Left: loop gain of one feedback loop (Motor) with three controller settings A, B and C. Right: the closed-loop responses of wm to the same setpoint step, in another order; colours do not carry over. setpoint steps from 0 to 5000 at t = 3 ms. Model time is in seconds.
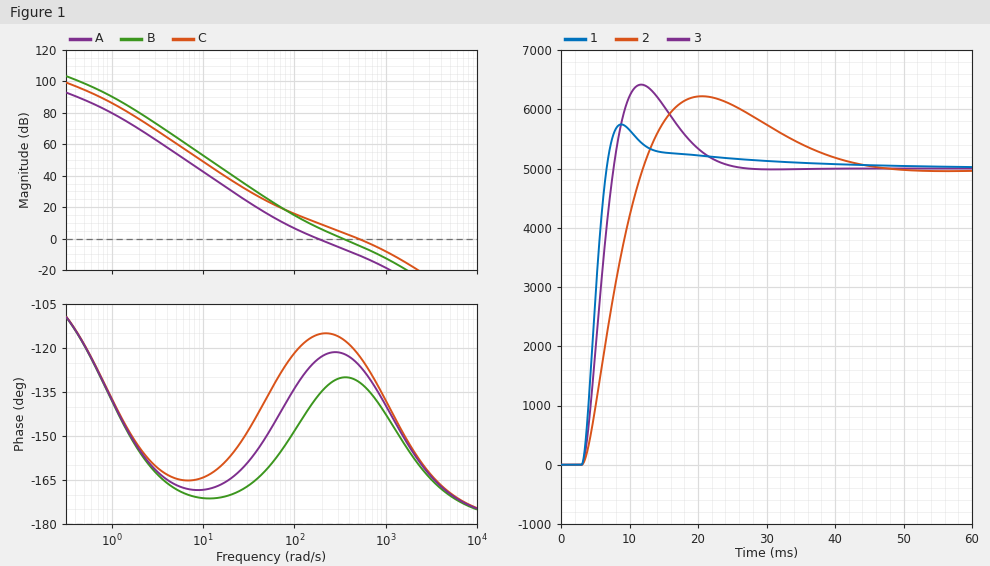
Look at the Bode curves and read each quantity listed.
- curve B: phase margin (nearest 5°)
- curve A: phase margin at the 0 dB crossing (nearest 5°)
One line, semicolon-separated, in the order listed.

50°; 55°
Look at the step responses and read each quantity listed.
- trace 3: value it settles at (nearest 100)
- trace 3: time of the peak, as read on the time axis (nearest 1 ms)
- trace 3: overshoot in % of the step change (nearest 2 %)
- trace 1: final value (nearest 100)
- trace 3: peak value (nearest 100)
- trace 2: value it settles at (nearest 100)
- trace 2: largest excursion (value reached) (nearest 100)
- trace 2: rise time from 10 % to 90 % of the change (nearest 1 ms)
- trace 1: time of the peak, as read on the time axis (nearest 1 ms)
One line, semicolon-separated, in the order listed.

5000; 12 ms; 28 %; 5000; 6400; 5000; 6200; 6 ms; 9 ms
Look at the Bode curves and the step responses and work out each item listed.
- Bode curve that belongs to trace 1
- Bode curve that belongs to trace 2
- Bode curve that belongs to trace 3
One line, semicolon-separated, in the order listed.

C; A; B
